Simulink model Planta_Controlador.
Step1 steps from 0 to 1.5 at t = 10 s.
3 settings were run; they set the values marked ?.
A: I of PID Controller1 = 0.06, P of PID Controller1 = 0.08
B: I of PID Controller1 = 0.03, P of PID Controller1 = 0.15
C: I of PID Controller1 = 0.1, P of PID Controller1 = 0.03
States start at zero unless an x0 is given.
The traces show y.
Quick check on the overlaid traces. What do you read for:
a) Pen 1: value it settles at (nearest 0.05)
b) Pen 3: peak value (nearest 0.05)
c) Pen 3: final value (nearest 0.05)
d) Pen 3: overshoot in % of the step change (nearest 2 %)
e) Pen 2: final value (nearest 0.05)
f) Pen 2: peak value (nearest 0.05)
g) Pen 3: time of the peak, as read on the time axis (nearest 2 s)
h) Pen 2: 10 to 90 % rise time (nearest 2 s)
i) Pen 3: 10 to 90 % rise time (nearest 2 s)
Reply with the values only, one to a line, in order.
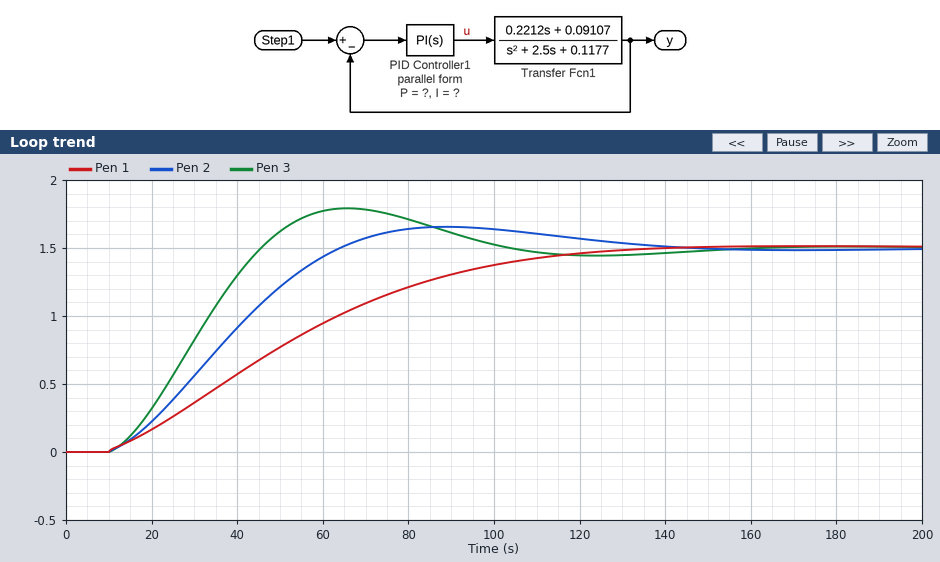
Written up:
1.50
1.80
1.50
20 %
1.50
1.65
66 s
38 s
26 s
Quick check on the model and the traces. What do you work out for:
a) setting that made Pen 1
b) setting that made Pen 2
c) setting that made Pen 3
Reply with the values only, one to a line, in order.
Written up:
B
A
C
